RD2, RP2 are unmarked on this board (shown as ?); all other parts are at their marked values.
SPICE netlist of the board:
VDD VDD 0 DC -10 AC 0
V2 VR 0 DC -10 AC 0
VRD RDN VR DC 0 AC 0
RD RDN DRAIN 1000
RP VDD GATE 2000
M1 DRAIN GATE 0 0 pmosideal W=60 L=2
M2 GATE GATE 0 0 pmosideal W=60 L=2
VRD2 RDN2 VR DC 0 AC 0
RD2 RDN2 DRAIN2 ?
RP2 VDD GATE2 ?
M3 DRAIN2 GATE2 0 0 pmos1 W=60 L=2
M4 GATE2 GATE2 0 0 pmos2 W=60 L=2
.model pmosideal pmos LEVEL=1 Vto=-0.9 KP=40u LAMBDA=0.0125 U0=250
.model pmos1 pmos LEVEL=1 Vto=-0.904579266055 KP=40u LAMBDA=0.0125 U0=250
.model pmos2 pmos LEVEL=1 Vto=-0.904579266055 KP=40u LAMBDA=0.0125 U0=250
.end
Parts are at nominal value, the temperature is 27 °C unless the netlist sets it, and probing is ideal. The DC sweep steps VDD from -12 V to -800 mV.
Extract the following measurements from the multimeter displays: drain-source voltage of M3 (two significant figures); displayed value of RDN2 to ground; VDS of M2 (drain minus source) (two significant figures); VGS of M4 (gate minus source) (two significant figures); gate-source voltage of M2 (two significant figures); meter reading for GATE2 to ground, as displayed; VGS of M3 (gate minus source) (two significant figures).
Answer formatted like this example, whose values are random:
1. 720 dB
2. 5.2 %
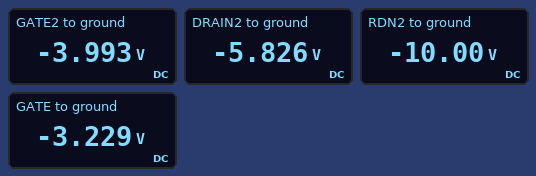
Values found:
1. -5.8 V
2. -10.00 V
3. -3.2 V
4. -4.0 V
5. -3.2 V
6. -3.993 V
7. -4.0 V
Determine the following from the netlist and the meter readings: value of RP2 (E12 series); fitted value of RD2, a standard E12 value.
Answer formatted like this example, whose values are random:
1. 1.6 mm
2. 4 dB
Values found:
1. 1 kΩ
2. 680 Ω
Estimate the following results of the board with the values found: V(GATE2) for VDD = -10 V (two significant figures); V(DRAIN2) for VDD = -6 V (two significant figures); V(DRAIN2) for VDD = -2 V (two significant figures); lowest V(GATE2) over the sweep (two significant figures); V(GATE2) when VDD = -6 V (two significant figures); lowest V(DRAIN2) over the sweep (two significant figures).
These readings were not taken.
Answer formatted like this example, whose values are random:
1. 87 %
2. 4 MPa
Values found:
1. -4.0 V
2. -7.9 V
3. -9.7 V
4. -4.4 V
5. -3.1 V
6. -10 V
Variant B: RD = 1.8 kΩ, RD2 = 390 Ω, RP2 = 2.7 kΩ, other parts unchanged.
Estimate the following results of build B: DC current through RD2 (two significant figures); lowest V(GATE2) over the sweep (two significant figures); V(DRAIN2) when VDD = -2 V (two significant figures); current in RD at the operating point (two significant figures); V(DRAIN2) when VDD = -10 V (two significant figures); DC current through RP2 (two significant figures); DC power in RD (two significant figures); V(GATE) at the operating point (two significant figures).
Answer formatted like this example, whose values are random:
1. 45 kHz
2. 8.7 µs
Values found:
1. 2.8 mA
2. -3.2 V
3. -9.9 V
4. 3.4 mA
5. -8.9 V
6. 2.6 mA
7. 21 mW
8. -3.2 V
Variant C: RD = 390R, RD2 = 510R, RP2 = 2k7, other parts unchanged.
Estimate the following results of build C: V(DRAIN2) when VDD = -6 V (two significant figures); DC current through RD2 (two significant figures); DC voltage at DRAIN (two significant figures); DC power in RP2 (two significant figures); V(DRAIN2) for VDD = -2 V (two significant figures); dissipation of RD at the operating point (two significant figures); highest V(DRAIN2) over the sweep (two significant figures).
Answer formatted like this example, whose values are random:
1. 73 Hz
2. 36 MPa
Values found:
1. -9.3 V
2. 2.8 mA
3. -8.6 V
4. 18 mW
5. -9.9 V
6. 5.1 mW
7. -8.2 V
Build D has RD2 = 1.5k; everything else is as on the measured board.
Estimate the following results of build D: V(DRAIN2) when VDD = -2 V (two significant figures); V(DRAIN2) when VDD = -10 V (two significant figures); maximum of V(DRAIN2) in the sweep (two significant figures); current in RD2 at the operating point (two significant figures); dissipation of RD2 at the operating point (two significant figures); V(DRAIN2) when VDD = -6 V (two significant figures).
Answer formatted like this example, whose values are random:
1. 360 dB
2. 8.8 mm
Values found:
1. -9.4 V
2. -2.1 V
3. -1.7 V
4. 5.3 mA
5. 42 mW
6. -5.5 V
